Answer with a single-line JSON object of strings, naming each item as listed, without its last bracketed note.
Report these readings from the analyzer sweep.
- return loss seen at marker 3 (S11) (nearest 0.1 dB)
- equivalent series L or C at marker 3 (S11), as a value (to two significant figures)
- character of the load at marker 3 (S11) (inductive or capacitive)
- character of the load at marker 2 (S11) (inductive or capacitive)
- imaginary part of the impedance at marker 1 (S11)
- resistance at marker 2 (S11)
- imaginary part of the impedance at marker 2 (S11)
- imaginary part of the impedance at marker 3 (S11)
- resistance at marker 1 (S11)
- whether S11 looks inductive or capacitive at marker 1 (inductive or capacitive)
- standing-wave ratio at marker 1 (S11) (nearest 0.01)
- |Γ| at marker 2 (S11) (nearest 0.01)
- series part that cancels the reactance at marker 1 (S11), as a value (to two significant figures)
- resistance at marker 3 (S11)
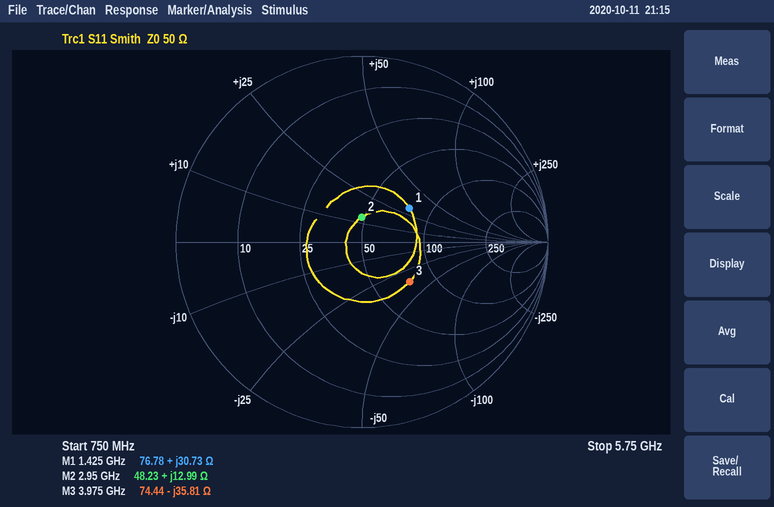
{"return loss seen at marker 3 (S11)": "9.5 dB", "equivalent series L or C at marker 3 (S11), as a value": "1.1 pF", "character of the load at marker 3 (S11)": "capacitive", "character of the load at marker 2 (S11)": "inductive", "imaginary part of the impedance at marker 1": "+30.73 Ω", "resistance at marker 2": "48.23 Ω", "imaginary part of the impedance at marker 2": "+12.99 Ω", "imaginary part of the impedance at marker 3": "-35.81 Ω", "resistance at marker 1": "76.78 Ω", "whether S11 looks inductive or capacitive at marker 1": "inductive", "standing-wave ratio at marker 1 (S11)": "1.91", "|Γ| at marker 2 (S11)": "0.13", "series part that cancels the reactance at marker 1 (S11), as a value": "3.6 pF", "resistance at marker 3": "74.44 Ω"}
